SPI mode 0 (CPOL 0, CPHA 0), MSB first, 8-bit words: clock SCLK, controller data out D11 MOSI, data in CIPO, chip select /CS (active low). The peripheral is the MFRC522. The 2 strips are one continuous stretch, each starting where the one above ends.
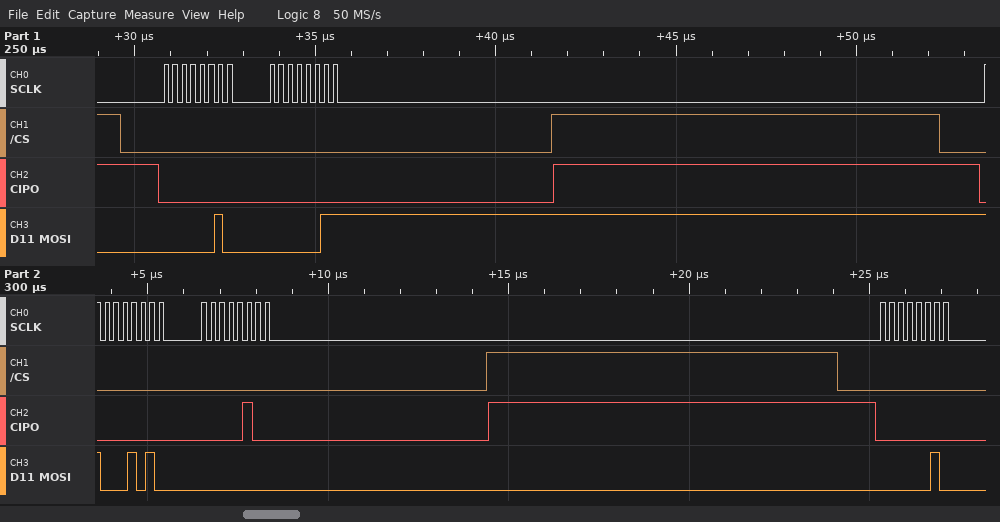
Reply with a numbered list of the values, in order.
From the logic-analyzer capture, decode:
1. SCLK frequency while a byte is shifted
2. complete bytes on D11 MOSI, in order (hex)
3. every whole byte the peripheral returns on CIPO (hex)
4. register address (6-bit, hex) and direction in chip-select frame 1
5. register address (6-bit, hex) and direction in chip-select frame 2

1. 4 MHz
2. 02 03 8A 00 02
3. 00 00 00 04 00
4. 0x01 write
5. 0x05 read
